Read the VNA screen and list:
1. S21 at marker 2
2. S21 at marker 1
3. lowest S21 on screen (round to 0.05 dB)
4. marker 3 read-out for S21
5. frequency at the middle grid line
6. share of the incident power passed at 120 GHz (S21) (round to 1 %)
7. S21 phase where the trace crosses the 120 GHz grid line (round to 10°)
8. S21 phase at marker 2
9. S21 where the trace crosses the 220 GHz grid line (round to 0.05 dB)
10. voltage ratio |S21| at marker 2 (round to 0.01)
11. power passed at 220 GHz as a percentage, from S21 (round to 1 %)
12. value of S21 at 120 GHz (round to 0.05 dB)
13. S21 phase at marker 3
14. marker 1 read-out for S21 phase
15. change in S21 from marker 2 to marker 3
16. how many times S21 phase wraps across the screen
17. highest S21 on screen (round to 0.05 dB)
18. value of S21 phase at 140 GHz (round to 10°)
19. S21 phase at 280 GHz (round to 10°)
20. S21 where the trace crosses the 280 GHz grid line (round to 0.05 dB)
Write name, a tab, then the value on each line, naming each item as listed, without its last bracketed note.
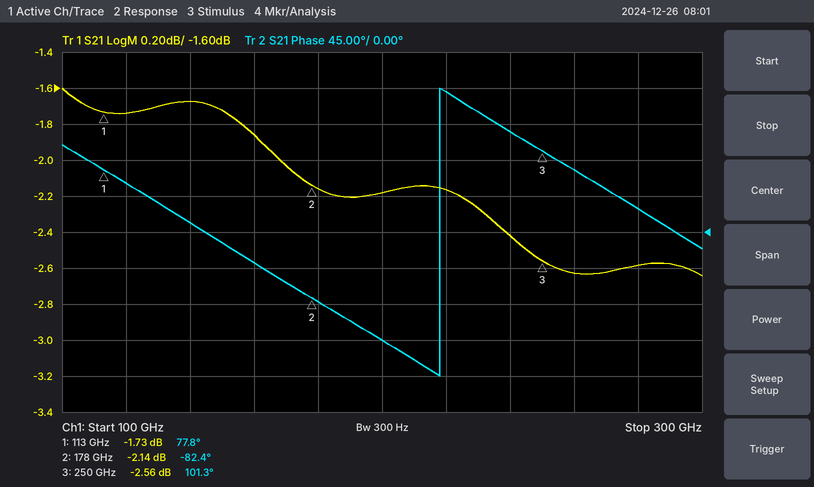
S21 at marker 2	-2.14 dB
S21 at marker 1	-1.73 dB
lowest S21 on screen	-2.65 dB
marker 3 read-out for S21	-2.56 dB
frequency at the middle grid line	200 GHz
share of the incident power passed at 120 GHz (S21)	67 %
S21 phase where the trace crosses the 120 GHz grid line	60°
S21 phase at marker 2	-82.4°
S21 where the trace crosses the 220 GHz grid line	-2.15 dB
voltage ratio |S21| at marker 2	0.78
power passed at 220 GHz as a percentage, from S21	61 %
value of S21 at 120 GHz	-1.75 dB
S21 phase at marker 3	101.3°
marker 1 read-out for S21 phase	77.8°
change in S21 from marker 2 to marker 3	-0.42 dB
how many times S21 phase wraps across the screen	1
highest S21 on screen	-1.60 dB
value of S21 phase at 140 GHz	10°
S21 phase at 280 GHz	30°
S21 where the trace crosses the 280 GHz grid line	-2.60 dB
